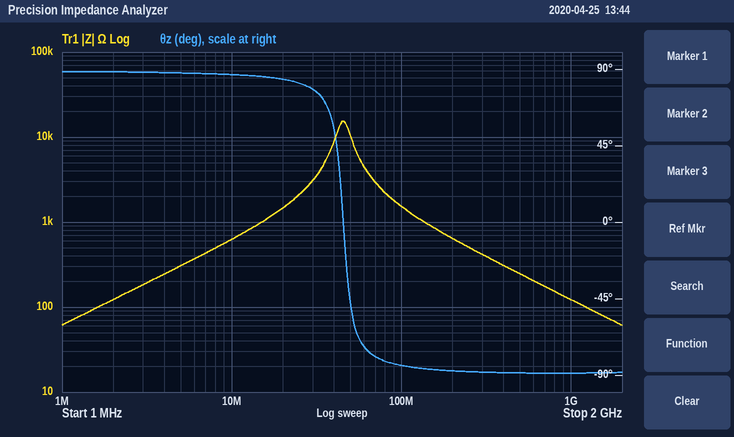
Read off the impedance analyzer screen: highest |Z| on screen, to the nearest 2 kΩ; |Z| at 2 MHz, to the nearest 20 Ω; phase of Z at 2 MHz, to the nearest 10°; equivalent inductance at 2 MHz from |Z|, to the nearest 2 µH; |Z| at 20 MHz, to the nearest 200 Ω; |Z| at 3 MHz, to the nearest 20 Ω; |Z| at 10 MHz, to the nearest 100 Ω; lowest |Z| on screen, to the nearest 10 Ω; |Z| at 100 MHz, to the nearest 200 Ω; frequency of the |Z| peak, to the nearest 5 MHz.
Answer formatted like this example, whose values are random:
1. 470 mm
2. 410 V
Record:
1. 16 kΩ
2. 120 Ω
3. 90°
4. 10 µH
5. 1.4 kΩ
6. 180 Ω
7. 600 Ω
8. 60 Ω
9. 1.6 kΩ
10. 45 MHz
